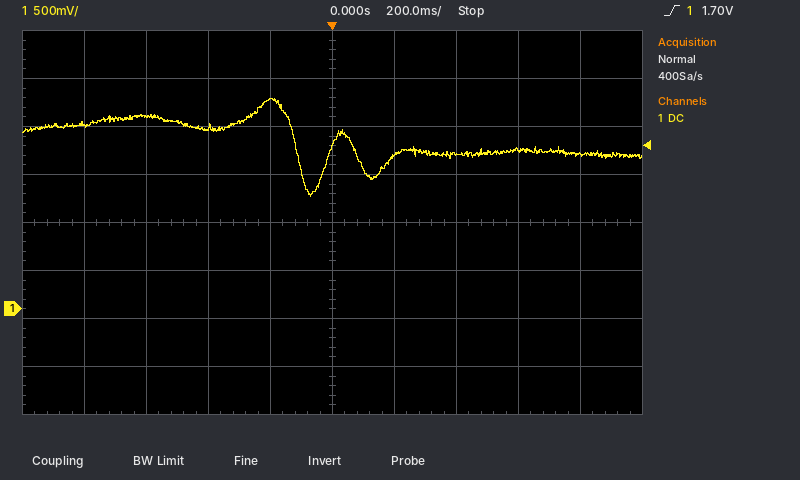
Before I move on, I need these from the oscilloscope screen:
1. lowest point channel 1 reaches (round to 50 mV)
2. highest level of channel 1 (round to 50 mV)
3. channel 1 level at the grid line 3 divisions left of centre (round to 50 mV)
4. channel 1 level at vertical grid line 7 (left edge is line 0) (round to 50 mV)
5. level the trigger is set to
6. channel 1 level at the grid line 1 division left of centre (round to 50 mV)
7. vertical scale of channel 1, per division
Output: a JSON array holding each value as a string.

["1.15 V", "2.20 V", "2.00 V", "1.60 V", "1.70 V", "2.20 V", "500 mV"]
